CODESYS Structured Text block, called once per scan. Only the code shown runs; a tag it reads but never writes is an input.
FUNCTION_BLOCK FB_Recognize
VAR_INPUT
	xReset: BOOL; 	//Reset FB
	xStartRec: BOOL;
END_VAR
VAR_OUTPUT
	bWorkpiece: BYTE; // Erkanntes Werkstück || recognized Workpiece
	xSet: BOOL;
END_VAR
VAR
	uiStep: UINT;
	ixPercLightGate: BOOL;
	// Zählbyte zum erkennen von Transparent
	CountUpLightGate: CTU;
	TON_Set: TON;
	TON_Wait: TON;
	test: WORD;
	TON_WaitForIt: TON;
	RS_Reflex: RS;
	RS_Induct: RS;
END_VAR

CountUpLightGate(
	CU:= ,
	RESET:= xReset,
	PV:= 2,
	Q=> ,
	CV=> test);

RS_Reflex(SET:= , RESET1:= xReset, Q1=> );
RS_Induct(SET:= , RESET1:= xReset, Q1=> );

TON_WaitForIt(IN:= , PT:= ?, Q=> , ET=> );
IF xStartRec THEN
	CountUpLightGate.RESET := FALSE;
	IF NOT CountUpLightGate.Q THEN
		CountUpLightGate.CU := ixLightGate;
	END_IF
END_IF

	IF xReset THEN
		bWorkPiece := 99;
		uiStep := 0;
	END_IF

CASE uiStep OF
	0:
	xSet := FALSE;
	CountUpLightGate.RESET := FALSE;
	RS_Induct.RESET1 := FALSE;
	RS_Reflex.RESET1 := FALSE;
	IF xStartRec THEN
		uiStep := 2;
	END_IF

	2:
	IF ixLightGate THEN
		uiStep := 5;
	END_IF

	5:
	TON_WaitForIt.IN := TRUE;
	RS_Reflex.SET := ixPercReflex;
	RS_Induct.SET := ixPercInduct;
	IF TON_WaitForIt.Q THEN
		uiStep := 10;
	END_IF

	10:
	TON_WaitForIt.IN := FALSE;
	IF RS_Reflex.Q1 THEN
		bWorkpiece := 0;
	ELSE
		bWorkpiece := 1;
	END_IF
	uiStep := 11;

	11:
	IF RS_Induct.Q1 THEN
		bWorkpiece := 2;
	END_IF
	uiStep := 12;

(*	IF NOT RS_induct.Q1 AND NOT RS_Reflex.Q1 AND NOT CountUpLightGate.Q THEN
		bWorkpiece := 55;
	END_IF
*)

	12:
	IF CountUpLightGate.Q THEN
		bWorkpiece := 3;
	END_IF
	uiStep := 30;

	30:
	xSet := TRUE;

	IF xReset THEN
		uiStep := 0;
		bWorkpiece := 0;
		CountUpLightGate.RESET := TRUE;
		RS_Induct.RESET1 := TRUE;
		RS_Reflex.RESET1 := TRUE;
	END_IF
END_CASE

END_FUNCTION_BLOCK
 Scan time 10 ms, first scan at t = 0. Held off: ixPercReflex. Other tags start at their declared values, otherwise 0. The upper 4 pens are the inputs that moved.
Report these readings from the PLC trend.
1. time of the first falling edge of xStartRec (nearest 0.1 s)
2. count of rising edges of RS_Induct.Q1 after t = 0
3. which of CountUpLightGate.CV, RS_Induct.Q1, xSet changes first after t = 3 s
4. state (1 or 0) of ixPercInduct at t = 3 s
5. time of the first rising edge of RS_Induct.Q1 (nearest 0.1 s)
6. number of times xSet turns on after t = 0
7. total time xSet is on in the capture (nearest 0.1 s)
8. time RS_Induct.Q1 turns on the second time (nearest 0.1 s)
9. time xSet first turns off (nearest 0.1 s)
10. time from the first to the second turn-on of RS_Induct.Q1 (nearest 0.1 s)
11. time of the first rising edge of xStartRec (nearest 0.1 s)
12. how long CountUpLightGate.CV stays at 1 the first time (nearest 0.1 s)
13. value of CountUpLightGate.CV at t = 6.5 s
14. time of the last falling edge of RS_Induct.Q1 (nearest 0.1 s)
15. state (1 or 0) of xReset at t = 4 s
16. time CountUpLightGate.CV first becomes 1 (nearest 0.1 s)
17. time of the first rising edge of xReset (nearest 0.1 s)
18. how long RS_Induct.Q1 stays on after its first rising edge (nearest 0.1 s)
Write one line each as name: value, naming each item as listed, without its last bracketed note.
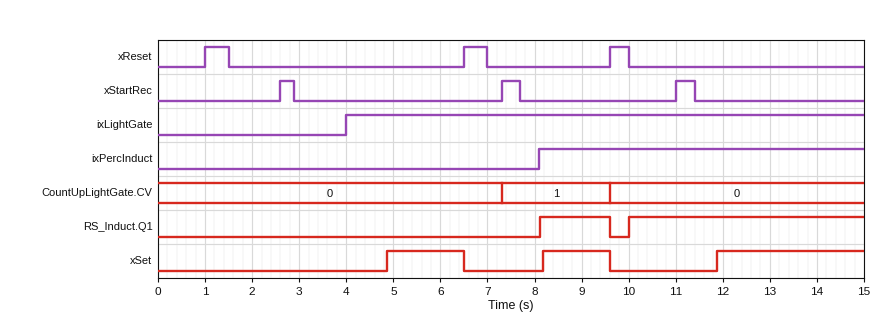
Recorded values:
time of the first falling edge of xStartRec: 2.9 s
count of rising edges of RS_Induct.Q1 after t = 0: 2
which of CountUpLightGate.CV, RS_Induct.Q1, xSet changes first after t = 3 s: xSet
state (1 or 0) of ixPercInduct at t = 3 s: 0
time of the first rising edge of RS_Induct.Q1: 8.1 s
number of times xSet turns on after t = 0: 3
total time xSet is on in the capture: 6.2 s
time RS_Induct.Q1 turns on the second time: 10.0 s
time xSet first turns off: 6.5 s
time from the first to the second turn-on of RS_Induct.Q1: 1.9 s
time of the first rising edge of xStartRec: 2.6 s
how long CountUpLightGate.CV stays at 1 the first time: 2.3 s
value of CountUpLightGate.CV at t = 6.5 s: 0
time of the last falling edge of RS_Induct.Q1: 9.6 s
state (1 or 0) of xReset at t = 4 s: 0
time CountUpLightGate.CV first becomes 1: 7.3 s
time of the first rising edge of xReset: 1.0 s
how long RS_Induct.Q1 stays on after its first rising edge: 1.5 s
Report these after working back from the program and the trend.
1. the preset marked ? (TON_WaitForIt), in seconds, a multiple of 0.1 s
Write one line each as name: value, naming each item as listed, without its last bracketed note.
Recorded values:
the preset marked ? (TON_WaitForIt), in seconds, a multiple of 0.1 s: 0.8 s
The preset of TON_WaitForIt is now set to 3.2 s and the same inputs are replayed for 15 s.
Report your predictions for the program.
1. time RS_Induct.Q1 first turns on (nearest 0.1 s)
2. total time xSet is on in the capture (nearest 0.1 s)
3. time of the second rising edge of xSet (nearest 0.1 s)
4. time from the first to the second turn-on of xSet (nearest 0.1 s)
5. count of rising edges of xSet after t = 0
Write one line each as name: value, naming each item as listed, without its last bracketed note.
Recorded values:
time RS_Induct.Q1 first turns on: 11.0 s
total time xSet is on in the capture: 3.0 s
time of the second rising edge of xSet: 14.3 s
time from the first to the second turn-on of xSet: 6.9 s
count of rising edges of xSet after t = 0: 2
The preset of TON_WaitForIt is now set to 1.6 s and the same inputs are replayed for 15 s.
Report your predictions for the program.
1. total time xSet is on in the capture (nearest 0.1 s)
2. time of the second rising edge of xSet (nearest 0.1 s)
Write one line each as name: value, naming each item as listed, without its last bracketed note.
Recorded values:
total time xSet is on in the capture: 3.8 s
time of the second rising edge of xSet: 9.0 s
